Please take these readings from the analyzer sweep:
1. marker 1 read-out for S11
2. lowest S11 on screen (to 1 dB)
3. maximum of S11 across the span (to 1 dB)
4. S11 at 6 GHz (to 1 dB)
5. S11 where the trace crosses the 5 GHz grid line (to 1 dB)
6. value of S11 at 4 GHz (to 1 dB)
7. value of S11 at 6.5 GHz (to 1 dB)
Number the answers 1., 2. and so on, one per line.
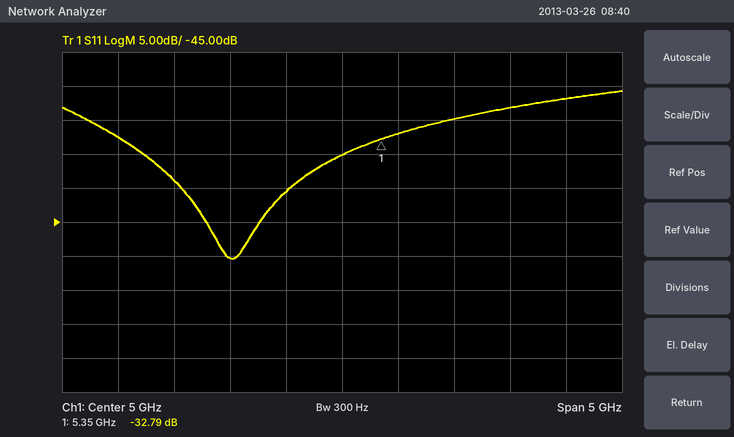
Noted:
1. -32.79 dB
2. -50 dB
3. -26 dB
4. -30 dB
5. -35 dB
6. -50 dB
7. -28 dB
